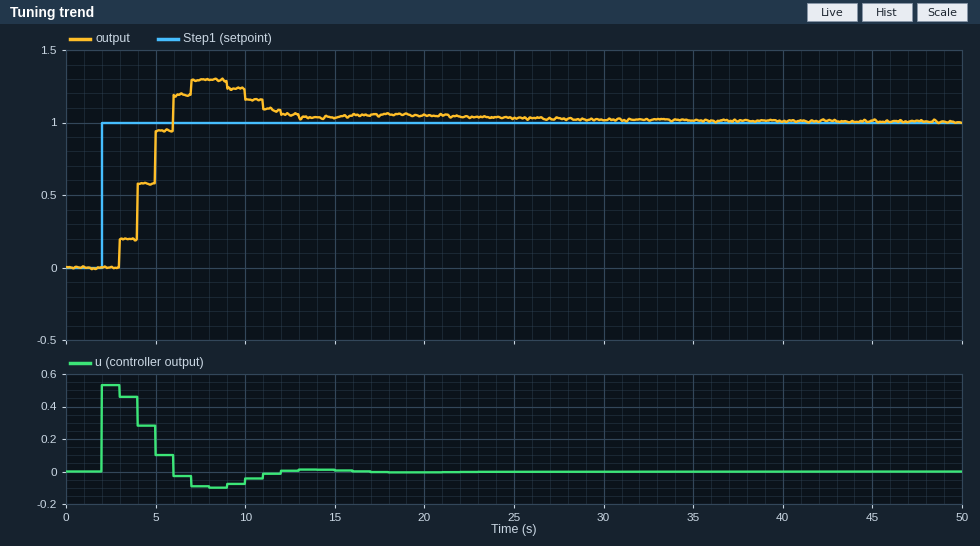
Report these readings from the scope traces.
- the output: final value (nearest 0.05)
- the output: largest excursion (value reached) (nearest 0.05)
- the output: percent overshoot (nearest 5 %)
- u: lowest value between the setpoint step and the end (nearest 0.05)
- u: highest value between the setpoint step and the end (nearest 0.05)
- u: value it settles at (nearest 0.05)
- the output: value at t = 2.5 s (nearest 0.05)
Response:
1.00
1.30
30 %
-0.10
0.55
0.00
0.00
